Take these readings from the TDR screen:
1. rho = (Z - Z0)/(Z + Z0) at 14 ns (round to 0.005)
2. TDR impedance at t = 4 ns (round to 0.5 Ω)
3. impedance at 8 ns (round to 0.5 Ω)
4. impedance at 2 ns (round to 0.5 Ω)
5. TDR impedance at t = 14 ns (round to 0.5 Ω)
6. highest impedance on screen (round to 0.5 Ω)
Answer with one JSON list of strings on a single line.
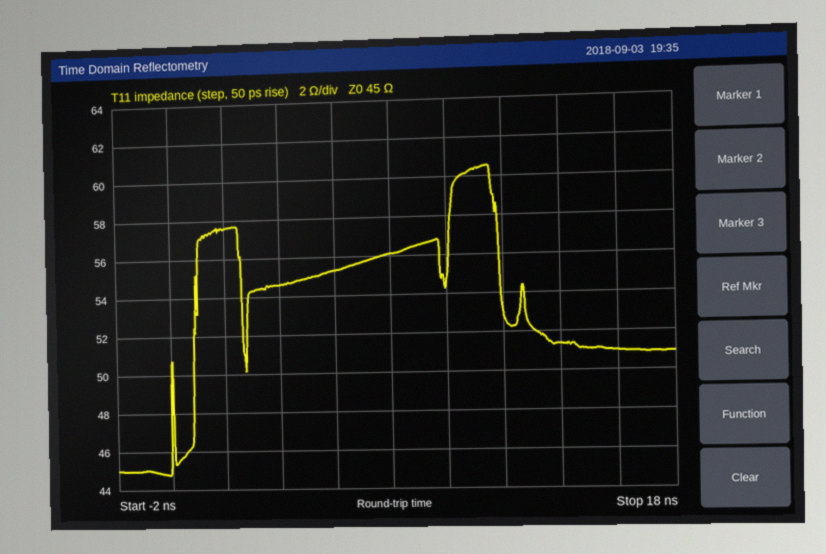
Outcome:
["+0.065", "54.5 Ω", "56.0 Ω", "57.5 Ω", "51.5 Ω", "60.5 Ω"]
